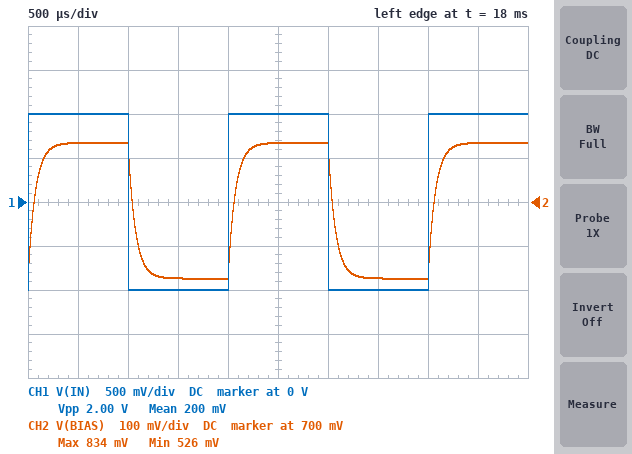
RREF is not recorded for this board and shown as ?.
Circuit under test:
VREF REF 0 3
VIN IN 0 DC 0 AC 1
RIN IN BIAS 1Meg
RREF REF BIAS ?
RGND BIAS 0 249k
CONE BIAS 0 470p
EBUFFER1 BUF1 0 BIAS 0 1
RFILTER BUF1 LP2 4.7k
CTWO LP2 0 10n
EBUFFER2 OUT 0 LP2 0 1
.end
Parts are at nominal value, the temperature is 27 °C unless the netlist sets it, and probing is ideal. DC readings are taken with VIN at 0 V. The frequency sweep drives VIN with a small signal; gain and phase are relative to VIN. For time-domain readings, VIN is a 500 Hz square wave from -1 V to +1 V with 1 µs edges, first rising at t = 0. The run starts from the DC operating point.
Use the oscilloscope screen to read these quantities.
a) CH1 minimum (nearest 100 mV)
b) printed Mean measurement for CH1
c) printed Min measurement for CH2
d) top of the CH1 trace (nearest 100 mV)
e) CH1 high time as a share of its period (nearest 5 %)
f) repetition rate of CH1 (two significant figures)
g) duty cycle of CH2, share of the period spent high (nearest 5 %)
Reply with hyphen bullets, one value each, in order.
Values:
- -1.0 V
- 200 mV
- 526 mV
- 1.0 V
- 50 %
- 500 Hz
- 50 %
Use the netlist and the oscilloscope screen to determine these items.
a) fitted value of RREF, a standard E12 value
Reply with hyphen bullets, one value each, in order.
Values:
- 680 kΩ
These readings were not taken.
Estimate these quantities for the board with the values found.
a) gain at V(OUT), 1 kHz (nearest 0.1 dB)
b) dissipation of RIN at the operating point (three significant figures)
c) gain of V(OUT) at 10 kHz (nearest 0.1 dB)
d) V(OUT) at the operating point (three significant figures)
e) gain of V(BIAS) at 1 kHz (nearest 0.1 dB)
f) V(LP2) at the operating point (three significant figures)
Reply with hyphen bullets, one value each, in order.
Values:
- -17.4 dB
- 463 nW
- -39.5 dB
- 680 mV
- -17.1 dB
- 680 mV
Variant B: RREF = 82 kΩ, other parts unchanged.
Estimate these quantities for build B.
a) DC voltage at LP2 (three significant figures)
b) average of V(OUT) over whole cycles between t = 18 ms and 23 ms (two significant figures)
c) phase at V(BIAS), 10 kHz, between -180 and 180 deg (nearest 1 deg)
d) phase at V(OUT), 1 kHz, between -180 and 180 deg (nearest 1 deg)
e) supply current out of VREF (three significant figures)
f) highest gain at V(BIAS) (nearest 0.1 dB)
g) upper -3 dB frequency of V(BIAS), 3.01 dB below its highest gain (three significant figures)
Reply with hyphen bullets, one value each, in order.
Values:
- 2.13 V
- 2.1 V
- -60 deg
- -26 deg
- 10.7 µA
- -24.7 dB
- 5.83 kHz
